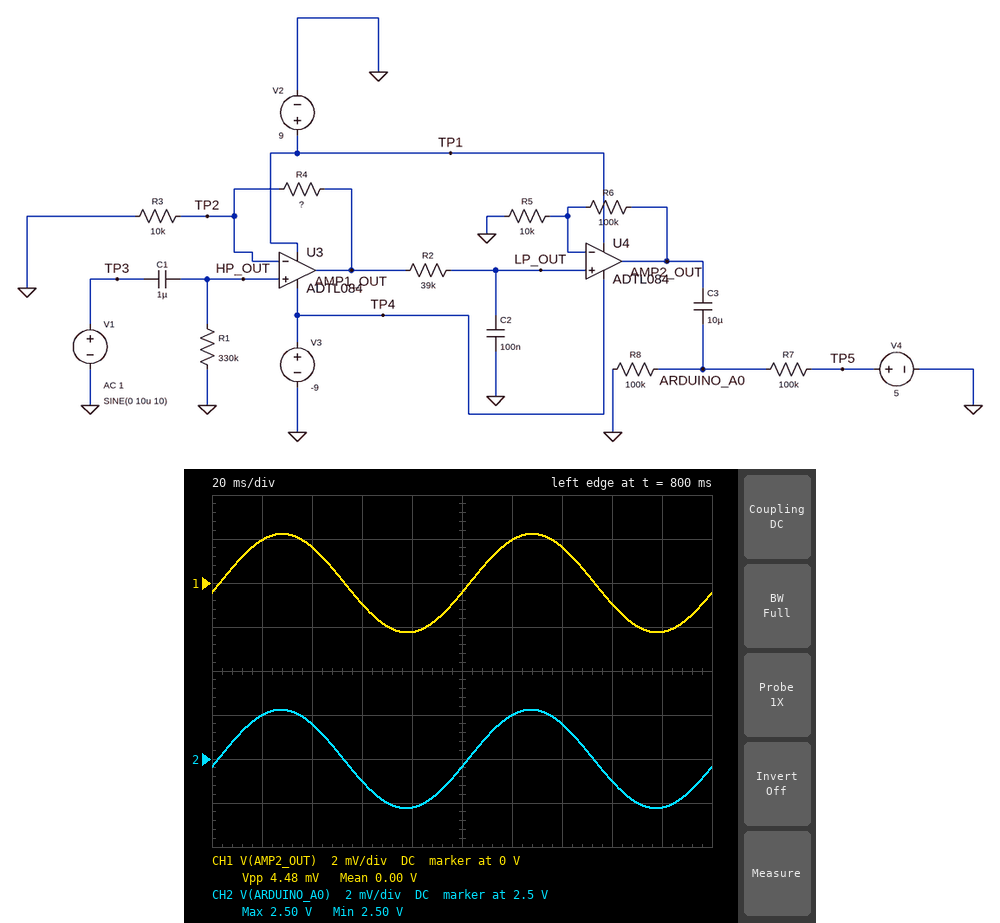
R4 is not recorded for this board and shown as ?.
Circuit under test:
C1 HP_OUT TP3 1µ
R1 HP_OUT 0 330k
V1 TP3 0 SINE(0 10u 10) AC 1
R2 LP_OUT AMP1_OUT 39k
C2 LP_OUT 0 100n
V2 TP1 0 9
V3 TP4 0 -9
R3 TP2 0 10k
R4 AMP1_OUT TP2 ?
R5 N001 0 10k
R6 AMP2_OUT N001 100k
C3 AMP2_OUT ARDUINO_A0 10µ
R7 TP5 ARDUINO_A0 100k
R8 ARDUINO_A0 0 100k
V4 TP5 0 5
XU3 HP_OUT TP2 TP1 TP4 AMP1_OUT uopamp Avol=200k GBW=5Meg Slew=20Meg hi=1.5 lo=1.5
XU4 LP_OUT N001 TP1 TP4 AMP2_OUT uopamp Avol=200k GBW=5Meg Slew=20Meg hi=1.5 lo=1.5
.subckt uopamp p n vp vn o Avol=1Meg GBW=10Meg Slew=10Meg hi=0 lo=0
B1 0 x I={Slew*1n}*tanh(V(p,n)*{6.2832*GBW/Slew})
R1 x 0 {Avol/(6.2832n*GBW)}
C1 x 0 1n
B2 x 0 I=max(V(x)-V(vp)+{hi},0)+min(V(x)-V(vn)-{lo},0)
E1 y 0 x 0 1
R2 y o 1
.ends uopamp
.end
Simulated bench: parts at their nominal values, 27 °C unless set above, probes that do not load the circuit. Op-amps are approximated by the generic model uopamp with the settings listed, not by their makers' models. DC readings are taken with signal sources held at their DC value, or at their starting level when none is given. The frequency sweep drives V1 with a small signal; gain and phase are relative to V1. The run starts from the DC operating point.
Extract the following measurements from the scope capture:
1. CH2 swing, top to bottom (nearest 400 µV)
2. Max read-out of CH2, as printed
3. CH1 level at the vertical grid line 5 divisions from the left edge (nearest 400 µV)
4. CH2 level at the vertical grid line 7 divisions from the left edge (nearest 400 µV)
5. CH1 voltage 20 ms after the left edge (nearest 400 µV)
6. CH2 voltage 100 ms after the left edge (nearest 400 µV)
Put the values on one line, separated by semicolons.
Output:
4.4 mV; 2.50 V; -400 µV; 2.5016 V; 2.0 mV; 2.4996 V
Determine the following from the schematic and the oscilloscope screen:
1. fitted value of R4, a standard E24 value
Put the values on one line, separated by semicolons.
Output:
200 kΩ
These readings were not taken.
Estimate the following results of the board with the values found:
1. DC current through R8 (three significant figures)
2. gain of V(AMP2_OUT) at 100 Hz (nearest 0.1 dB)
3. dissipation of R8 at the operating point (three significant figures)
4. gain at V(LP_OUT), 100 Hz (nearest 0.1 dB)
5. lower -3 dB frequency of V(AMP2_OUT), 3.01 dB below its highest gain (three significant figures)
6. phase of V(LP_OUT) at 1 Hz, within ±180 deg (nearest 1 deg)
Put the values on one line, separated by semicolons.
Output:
25.0 µA; 38.8 dB; 62.5 µW; 18.0 dB; 471 mHz; 24 deg
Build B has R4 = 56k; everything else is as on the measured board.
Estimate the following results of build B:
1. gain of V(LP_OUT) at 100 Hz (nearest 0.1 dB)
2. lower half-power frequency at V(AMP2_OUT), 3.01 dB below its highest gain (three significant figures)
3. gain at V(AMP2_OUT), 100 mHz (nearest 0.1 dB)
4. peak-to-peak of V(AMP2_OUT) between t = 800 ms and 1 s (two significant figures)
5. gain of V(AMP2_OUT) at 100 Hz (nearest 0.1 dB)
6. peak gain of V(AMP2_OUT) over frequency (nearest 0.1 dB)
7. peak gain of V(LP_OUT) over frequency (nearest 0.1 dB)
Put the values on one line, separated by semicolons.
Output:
7.9 dB; 471 mHz; 23.4 dB; 1.4 mV; 28.8 dB; 37.1 dB; 16.3 dB
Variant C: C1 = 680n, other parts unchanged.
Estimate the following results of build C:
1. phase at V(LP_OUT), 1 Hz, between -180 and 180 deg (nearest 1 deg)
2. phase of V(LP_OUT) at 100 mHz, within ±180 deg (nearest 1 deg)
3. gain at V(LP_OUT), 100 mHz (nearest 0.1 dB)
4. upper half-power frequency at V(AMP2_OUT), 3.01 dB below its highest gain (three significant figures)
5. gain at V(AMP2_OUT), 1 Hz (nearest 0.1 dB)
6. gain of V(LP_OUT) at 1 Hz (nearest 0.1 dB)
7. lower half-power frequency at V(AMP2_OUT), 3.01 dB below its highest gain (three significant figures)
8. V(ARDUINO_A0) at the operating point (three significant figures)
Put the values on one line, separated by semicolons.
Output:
34 deg; 82 deg; 9.3 dB; 42.2 Hz; 45.5 dB; 24.7 dB; 686 mHz; 2.50 V
